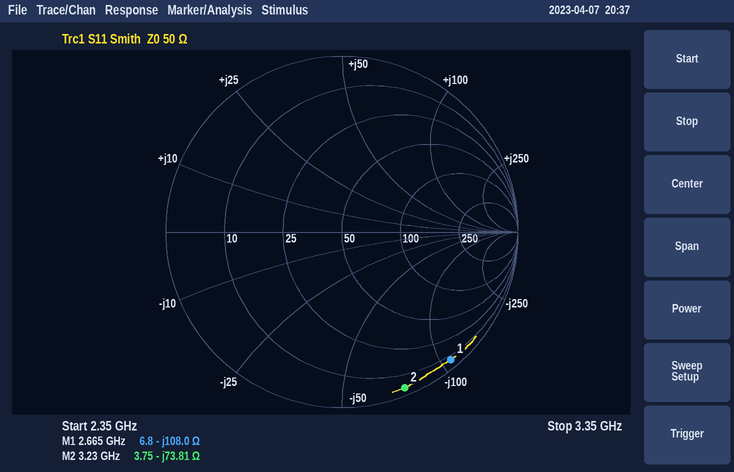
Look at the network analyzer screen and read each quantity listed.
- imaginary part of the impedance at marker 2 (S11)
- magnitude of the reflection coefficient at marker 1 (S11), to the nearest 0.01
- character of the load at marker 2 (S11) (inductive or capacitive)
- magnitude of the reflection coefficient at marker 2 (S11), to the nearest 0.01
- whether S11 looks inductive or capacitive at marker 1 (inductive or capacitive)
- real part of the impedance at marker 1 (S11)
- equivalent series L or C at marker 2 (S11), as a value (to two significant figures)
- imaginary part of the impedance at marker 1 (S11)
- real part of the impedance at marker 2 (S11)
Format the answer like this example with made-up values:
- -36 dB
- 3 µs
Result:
- -73.81 Ω
- 0.95
- capacitive
- 0.95
- capacitive
- 6.8 Ω
- 670 fF
- -108.0 Ω
- 3.75 Ω
